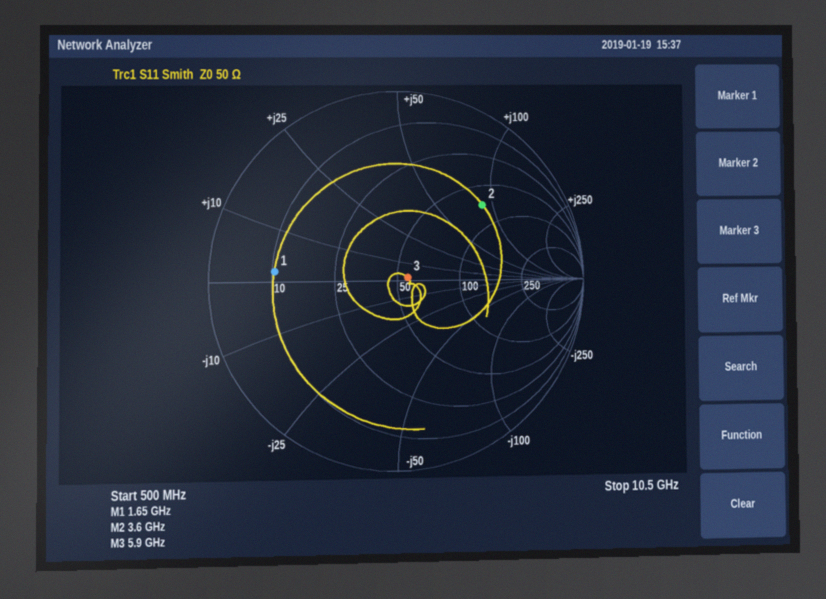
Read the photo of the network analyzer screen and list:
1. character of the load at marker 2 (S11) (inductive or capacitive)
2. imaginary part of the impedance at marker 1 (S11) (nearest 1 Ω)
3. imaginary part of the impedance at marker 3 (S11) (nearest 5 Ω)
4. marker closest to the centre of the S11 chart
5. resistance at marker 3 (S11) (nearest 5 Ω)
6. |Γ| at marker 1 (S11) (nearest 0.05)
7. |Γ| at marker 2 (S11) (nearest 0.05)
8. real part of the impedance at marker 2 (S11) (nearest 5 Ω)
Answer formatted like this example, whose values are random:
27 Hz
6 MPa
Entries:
inductive
+2 Ω
0 Ω
marker 3
55 Ω
0.65
0.60
70 Ω
